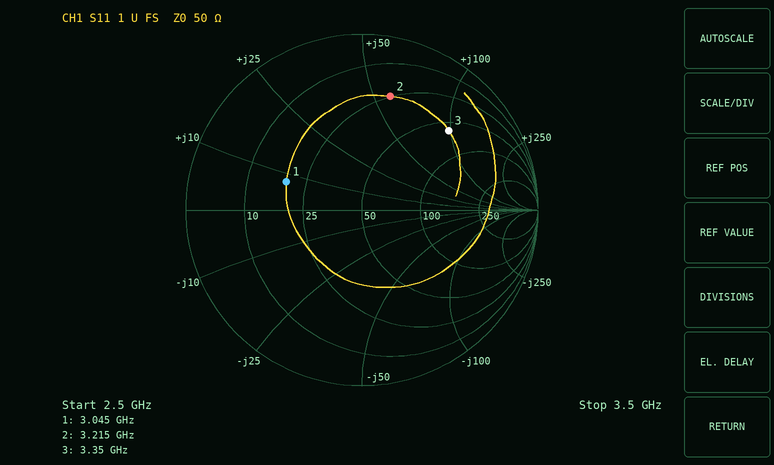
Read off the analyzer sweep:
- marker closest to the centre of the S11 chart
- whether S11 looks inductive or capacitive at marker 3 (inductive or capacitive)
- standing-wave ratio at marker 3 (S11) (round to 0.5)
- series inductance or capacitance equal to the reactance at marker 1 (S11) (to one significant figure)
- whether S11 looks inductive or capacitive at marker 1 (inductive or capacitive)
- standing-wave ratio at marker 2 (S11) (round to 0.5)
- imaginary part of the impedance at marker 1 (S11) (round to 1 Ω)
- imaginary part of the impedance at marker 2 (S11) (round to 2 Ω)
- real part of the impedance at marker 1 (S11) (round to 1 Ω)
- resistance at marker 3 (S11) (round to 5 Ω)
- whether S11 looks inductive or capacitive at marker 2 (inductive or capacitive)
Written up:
marker 1
inductive
5.0
400 pH
inductive
5.0
+8 Ω
+58 Ω
19 Ω
60 Ω
inductive
